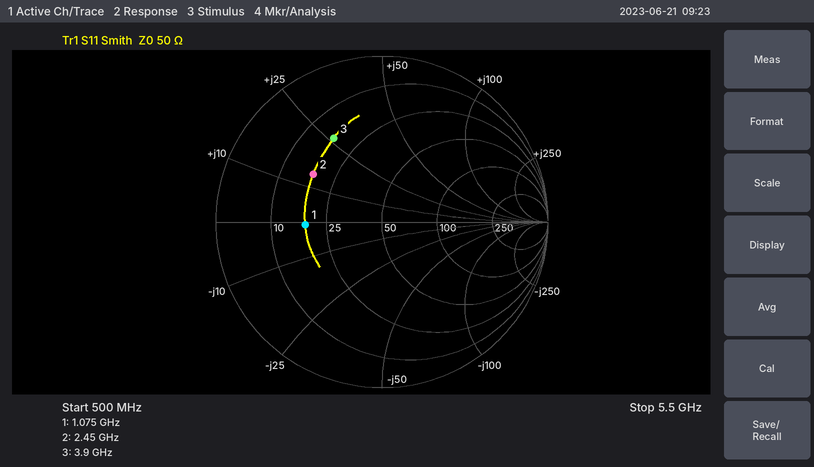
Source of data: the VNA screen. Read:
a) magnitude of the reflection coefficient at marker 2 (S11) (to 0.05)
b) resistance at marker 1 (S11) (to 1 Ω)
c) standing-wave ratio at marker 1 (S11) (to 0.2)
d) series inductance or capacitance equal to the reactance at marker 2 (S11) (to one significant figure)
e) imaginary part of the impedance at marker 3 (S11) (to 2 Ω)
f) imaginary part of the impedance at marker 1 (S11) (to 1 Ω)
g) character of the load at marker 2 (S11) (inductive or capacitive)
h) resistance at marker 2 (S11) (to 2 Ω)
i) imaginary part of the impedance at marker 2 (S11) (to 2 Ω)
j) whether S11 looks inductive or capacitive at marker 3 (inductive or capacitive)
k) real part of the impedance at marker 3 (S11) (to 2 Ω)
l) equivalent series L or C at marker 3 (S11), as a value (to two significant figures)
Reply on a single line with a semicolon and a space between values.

0.50; 18 Ω; 2.8; 900 pH; +26 Ω; -1 Ω; inductive; 18 Ω; +14 Ω; inductive; 18 Ω; 1.1 nH
